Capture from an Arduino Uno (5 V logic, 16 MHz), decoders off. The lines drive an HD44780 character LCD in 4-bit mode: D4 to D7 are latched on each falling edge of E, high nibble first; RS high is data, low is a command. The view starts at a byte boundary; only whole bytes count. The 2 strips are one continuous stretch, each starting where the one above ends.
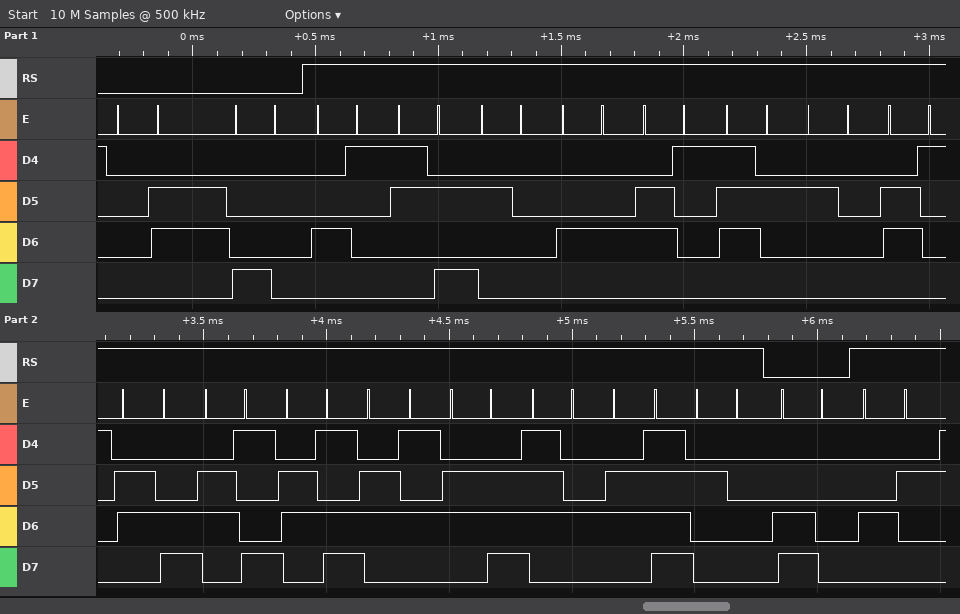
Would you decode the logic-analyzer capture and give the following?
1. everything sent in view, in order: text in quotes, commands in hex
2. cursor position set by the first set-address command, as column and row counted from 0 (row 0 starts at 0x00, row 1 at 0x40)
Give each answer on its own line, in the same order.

0x06 0x80 "A: Dar alimento " 0xC0 "B"
column 0, row 0
